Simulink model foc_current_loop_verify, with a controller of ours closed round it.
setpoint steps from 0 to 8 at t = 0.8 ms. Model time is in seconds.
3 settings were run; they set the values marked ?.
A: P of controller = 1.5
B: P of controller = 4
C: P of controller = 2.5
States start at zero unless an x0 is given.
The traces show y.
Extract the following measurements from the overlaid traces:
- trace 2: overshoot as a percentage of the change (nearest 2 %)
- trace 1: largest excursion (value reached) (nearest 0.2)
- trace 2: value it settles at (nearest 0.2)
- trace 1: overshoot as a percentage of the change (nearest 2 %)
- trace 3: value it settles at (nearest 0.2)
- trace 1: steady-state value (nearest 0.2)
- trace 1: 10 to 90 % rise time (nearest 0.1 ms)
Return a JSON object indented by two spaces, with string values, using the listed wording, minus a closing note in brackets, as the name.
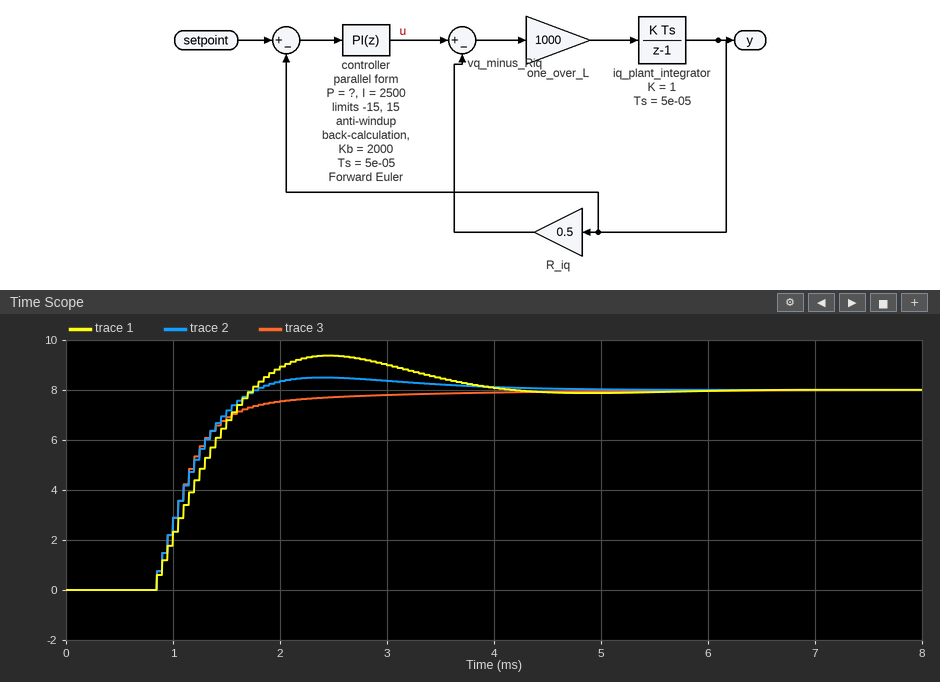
{
  "trace 2: overshoot as a percentage of the change": "6 %",
  "trace 1: largest excursion (value reached)": "9.4",
  "trace 2: value it settles at": "8.0",
  "trace 1: overshoot as a percentage of the change": "18 %",
  "trace 3: value it settles at": "8.0",
  "trace 1: steady-state value": "8.0",
  "trace 1: 10 to 90 % rise time": "0.7 ms"
}
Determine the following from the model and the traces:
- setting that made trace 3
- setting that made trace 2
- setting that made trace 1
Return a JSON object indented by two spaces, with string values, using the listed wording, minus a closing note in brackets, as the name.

{
  "setting that made trace 3": "B",
  "setting that made trace 2": "C",
  "setting that made trace 1": "A"
}
